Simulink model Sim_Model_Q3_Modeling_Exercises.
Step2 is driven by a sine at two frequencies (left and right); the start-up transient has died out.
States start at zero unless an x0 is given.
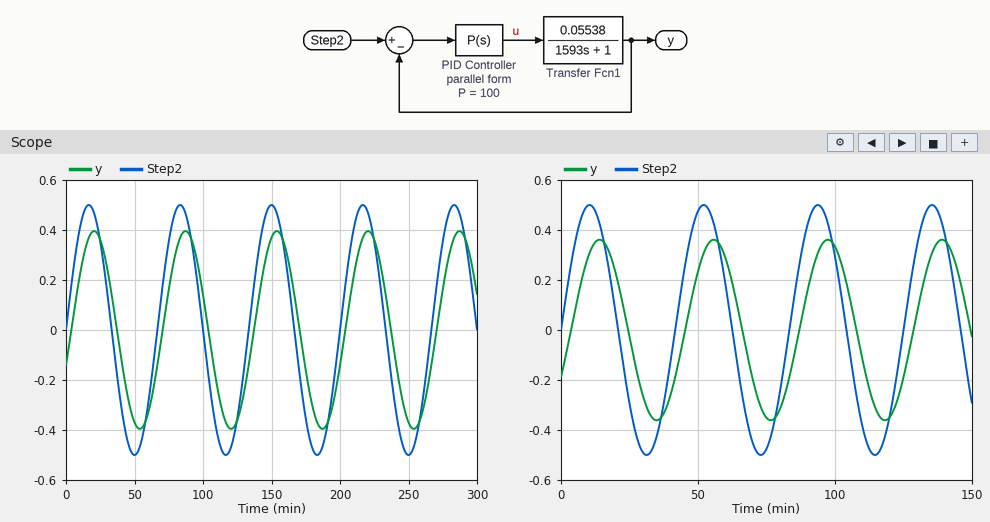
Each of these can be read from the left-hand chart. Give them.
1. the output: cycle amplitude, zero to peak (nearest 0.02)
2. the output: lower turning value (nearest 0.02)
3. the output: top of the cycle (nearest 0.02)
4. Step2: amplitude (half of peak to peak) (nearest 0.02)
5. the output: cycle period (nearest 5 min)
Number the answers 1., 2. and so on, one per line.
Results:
1. 0.40
2. -0.40
3. 0.40
4. 0.50
5. 65 min
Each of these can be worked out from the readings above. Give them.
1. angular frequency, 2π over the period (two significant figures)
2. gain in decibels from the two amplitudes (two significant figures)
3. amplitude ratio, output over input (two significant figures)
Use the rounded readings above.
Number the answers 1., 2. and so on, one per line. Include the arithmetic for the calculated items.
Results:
1. 2π / 65 = 0.097 rad/min
2. 20 log10(0.4 / 0.5) = -1.9 dB
3. 0.4 / 0.5 = 0.80
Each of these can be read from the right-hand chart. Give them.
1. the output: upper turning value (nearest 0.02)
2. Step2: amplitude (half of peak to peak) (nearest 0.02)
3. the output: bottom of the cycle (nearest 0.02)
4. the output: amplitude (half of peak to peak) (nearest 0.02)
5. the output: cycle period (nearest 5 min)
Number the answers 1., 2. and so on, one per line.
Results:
1. 0.36
2. 0.50
3. -0.36
4. 0.36
5. 40 min
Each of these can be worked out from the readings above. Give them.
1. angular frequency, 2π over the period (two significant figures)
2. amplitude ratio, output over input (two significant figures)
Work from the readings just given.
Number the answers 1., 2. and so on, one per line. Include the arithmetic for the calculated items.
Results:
1. 2π / 40 = 0.16 rad/min
2. 0.36 / 0.5 = 0.72
